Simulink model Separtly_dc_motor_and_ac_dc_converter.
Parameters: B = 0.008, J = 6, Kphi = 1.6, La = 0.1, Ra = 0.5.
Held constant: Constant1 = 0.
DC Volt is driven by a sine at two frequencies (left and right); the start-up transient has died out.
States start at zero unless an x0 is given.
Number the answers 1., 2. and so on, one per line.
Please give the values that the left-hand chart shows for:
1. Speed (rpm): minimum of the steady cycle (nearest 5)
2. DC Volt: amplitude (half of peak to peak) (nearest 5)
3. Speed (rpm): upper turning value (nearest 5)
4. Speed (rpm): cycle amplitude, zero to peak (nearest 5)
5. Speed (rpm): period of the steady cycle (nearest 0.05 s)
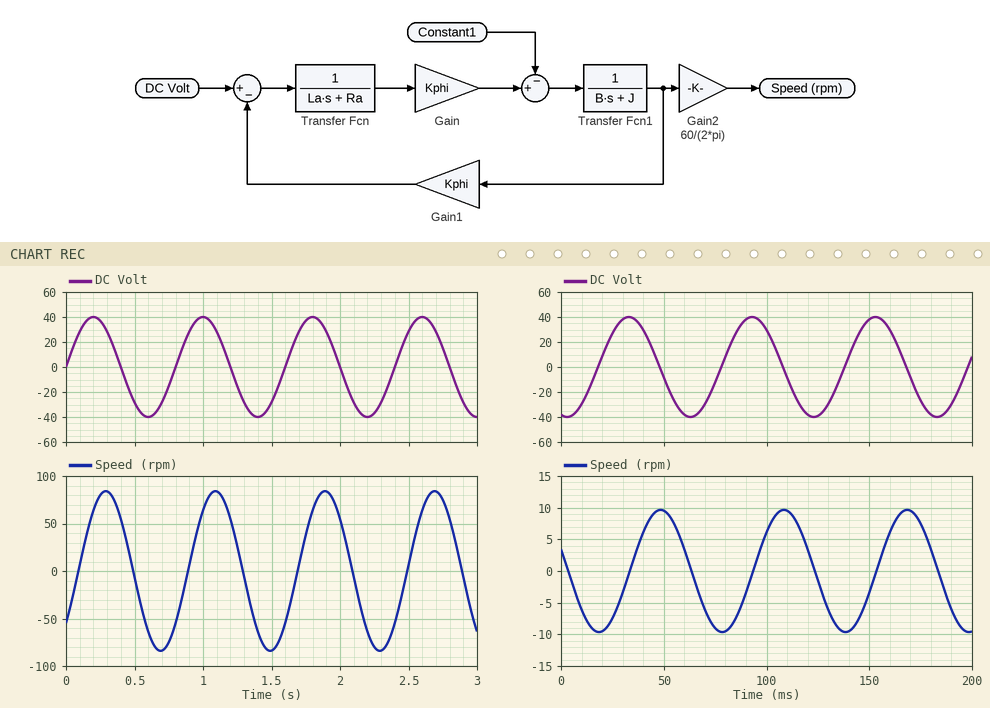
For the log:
1. -85
2. 40
3. 85
4. 85
5. 0.80 s
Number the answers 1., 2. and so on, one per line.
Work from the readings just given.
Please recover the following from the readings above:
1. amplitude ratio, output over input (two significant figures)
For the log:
1. 2.1
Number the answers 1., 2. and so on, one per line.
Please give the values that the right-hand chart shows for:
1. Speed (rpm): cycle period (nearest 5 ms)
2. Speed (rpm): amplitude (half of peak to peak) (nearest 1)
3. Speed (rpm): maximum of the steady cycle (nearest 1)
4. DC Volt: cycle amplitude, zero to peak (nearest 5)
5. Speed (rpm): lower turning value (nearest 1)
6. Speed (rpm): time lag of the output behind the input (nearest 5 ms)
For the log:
1. 60 ms
2. 10
3. 10
4. 40
5. -10
6. 15 ms
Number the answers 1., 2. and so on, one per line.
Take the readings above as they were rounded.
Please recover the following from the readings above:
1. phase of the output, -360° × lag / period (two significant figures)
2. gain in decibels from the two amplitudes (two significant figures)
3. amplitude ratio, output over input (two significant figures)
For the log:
1. -90°
2. -12 dB
3. 0.25
